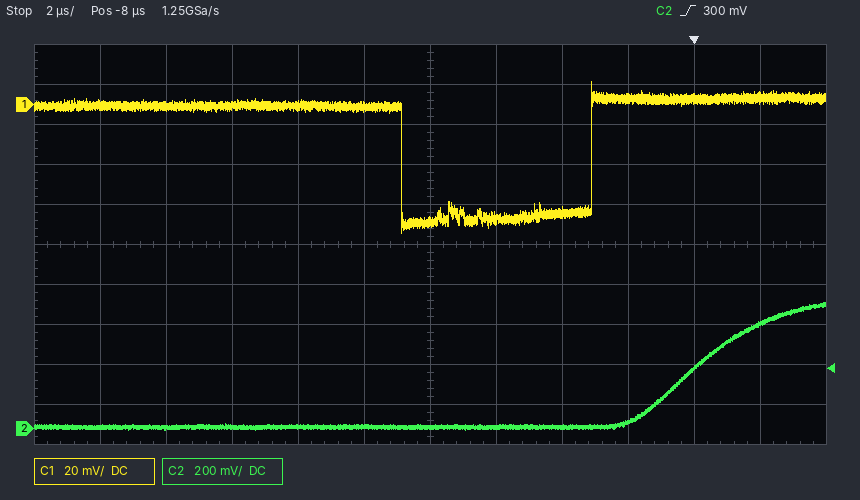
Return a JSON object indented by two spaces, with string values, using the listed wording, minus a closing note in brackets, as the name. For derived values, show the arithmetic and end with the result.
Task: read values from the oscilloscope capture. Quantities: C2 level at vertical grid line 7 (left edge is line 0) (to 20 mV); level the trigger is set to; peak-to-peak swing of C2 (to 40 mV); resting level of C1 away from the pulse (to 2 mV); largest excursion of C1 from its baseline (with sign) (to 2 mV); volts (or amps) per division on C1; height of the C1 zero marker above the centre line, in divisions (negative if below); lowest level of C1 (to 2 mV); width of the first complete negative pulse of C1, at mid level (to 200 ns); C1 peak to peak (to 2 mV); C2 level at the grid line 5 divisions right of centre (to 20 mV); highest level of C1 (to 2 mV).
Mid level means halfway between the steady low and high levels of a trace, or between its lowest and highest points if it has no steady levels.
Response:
{
  "C2 level at vertical grid line 7 (left edge is line 0)": "0 mV",
  "level the trigger is set to": "300 mV",
  "peak-to-peak swing of C2": "640 mV",
  "resting level of C1 away from the pulse": "0 mV",
  "largest excursion of C1 from its baseline (with sign)": "-64 mV − (0 mV) = -64 mV",
  "volts (or amps) per division on C1": "20 mV",
  "height of the C1 zero marker above the centre line, in divisions": "+3.5 div",
  "lowest level of C1": "-64 mV",
  "width of the first complete negative pulse of C1, at mid level": "5.8 µs",
  "C1 peak to peak": "12 mV − (-64 mV) = 76 mV",
  "C2 level at the grid line 5 divisions right of centre": "520 mV",
  "highest level of C1": "12 mV"
}
